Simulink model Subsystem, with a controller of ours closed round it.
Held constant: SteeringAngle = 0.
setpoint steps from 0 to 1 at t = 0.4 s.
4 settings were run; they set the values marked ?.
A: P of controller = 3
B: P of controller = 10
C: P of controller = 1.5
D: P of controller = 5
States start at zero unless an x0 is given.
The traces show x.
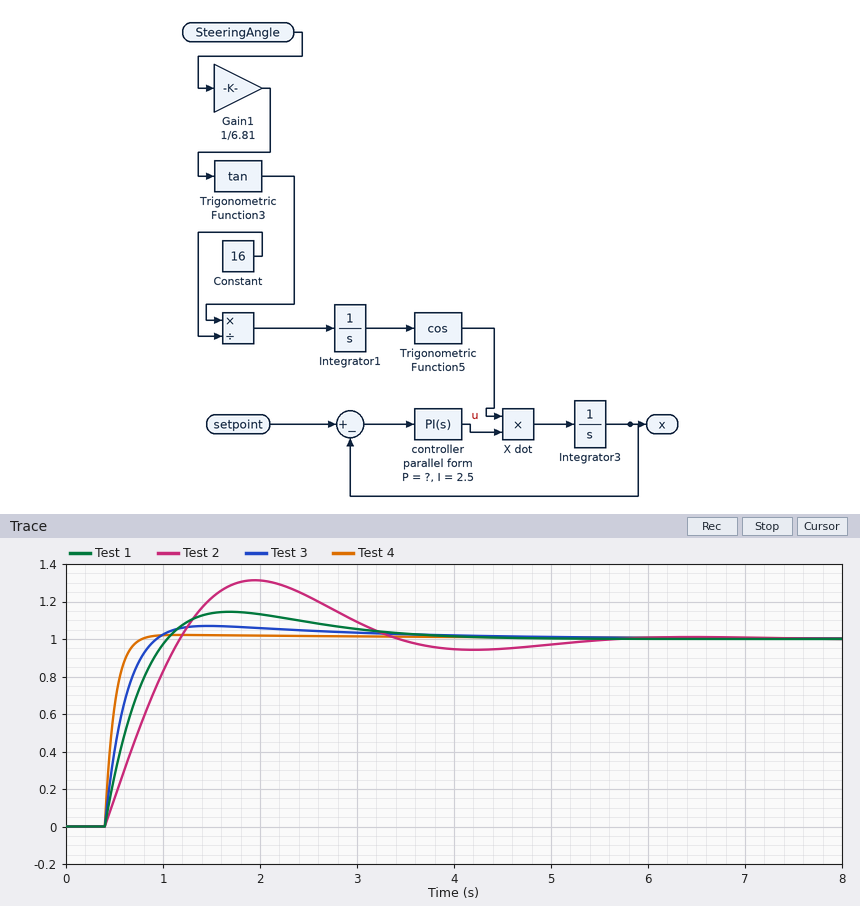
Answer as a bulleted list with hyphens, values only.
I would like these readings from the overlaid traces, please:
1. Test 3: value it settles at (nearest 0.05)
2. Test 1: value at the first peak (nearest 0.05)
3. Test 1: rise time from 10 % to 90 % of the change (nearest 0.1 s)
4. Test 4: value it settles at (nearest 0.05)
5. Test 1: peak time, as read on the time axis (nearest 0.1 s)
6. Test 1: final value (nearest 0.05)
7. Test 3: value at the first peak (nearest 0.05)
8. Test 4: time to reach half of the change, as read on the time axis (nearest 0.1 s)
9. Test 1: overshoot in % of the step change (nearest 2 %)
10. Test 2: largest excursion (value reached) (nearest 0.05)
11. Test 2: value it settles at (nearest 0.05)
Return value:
- 1.00
- 1.15
- 0.5 s
- 1.00
- 1.7 s
- 1.00
- 1.05
- 0.5 s
- 14 %
- 1.30
- 1.00
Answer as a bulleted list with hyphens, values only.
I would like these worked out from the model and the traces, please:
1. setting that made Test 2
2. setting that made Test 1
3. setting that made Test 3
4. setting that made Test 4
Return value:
- C
- A
- D
- B
